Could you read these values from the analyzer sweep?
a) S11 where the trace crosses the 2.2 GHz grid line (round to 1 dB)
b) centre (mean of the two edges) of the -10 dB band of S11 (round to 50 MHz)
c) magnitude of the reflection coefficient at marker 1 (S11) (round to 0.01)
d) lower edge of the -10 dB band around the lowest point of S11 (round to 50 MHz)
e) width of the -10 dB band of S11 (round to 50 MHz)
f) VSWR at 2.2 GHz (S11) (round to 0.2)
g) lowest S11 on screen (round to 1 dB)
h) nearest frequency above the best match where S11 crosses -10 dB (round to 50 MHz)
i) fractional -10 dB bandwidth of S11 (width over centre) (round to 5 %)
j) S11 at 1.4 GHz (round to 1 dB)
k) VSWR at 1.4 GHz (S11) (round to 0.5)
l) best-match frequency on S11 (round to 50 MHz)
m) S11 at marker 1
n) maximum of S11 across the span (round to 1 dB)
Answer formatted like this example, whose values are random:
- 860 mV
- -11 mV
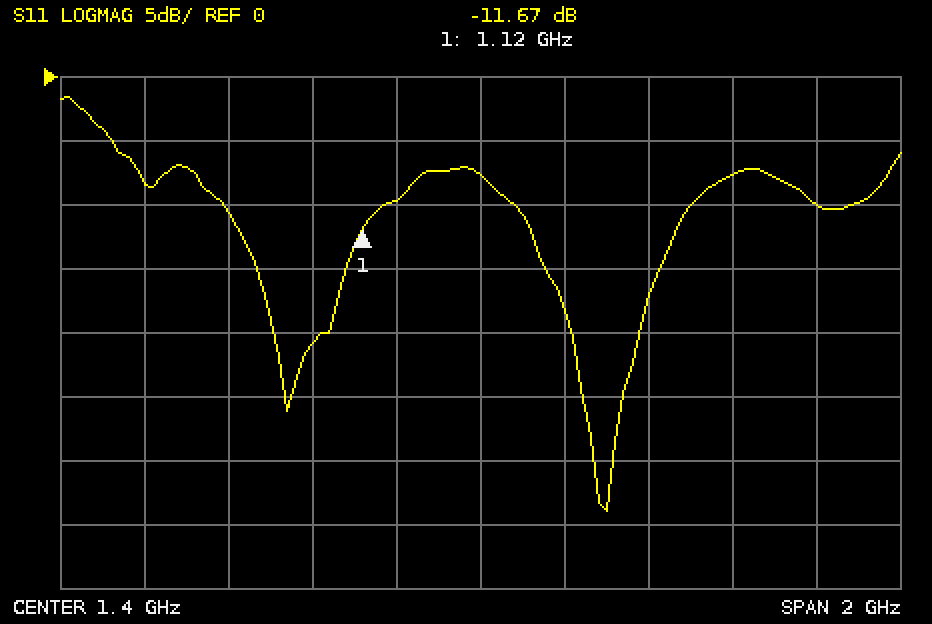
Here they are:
- -10 dB
- 1.70 GHz
- 0.26
- 1.50 GHz
- 400 MHz
- 2.0
- -34 dB
- 1.90 GHz
- 25 %
- -8 dB
- 2.5
- 1.70 GHz
- -11.67 dB
- -2 dB
